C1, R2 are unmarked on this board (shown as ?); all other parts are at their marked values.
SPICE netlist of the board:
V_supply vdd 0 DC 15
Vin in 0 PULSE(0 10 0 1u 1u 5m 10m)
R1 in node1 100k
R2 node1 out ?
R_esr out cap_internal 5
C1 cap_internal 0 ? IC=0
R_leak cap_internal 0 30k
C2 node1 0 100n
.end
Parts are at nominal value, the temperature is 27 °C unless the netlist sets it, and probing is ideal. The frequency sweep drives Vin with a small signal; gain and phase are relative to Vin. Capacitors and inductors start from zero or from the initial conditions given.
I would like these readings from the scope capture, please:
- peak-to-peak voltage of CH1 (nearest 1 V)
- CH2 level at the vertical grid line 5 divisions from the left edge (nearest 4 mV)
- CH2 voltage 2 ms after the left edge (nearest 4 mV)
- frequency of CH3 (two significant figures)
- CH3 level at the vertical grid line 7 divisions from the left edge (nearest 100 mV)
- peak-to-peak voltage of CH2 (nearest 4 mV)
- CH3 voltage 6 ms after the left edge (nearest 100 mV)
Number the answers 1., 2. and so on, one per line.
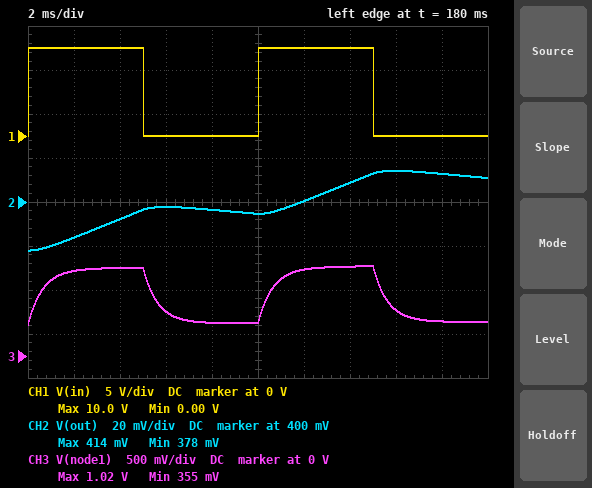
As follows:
1. 10 V
2. 396 mV
3. 384 mV
4. 100 Hz
5. 1.0 V
6. 36 mV
7. 500 mV
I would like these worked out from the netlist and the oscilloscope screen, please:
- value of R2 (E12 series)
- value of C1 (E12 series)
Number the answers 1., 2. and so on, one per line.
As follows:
1. 6.8 kΩ
2. 18 µF
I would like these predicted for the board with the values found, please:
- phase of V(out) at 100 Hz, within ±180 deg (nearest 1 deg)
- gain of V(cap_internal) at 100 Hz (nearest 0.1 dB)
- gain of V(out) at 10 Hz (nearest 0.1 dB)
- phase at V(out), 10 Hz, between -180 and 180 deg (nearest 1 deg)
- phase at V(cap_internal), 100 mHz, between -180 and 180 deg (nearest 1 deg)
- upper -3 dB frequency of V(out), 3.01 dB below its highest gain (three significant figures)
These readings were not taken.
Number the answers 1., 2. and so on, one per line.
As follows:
1. -108 deg
2. -62.3 dB
3. -41.7 dB
4. -90 deg
5. -15 deg
6. 376 mHz
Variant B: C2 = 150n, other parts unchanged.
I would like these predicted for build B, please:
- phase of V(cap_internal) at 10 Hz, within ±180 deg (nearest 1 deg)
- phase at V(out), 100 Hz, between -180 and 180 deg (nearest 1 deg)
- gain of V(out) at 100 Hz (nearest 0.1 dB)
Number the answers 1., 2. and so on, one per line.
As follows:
1. -91 deg
2. -117 deg
3. -63.0 dB
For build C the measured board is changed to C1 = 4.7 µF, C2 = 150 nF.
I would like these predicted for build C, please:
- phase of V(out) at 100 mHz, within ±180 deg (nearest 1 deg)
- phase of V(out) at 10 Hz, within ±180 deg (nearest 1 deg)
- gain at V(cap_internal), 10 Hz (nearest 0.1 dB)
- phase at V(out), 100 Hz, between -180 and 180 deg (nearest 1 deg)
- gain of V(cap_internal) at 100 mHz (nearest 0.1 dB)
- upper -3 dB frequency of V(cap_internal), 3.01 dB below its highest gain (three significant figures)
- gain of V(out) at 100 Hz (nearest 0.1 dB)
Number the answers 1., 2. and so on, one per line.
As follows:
1. -4 deg
2. -85 deg
3. -30.3 dB
4. -119 deg
5. -13.2 dB
6. 1.41 Hz
7. -51.5 dB
